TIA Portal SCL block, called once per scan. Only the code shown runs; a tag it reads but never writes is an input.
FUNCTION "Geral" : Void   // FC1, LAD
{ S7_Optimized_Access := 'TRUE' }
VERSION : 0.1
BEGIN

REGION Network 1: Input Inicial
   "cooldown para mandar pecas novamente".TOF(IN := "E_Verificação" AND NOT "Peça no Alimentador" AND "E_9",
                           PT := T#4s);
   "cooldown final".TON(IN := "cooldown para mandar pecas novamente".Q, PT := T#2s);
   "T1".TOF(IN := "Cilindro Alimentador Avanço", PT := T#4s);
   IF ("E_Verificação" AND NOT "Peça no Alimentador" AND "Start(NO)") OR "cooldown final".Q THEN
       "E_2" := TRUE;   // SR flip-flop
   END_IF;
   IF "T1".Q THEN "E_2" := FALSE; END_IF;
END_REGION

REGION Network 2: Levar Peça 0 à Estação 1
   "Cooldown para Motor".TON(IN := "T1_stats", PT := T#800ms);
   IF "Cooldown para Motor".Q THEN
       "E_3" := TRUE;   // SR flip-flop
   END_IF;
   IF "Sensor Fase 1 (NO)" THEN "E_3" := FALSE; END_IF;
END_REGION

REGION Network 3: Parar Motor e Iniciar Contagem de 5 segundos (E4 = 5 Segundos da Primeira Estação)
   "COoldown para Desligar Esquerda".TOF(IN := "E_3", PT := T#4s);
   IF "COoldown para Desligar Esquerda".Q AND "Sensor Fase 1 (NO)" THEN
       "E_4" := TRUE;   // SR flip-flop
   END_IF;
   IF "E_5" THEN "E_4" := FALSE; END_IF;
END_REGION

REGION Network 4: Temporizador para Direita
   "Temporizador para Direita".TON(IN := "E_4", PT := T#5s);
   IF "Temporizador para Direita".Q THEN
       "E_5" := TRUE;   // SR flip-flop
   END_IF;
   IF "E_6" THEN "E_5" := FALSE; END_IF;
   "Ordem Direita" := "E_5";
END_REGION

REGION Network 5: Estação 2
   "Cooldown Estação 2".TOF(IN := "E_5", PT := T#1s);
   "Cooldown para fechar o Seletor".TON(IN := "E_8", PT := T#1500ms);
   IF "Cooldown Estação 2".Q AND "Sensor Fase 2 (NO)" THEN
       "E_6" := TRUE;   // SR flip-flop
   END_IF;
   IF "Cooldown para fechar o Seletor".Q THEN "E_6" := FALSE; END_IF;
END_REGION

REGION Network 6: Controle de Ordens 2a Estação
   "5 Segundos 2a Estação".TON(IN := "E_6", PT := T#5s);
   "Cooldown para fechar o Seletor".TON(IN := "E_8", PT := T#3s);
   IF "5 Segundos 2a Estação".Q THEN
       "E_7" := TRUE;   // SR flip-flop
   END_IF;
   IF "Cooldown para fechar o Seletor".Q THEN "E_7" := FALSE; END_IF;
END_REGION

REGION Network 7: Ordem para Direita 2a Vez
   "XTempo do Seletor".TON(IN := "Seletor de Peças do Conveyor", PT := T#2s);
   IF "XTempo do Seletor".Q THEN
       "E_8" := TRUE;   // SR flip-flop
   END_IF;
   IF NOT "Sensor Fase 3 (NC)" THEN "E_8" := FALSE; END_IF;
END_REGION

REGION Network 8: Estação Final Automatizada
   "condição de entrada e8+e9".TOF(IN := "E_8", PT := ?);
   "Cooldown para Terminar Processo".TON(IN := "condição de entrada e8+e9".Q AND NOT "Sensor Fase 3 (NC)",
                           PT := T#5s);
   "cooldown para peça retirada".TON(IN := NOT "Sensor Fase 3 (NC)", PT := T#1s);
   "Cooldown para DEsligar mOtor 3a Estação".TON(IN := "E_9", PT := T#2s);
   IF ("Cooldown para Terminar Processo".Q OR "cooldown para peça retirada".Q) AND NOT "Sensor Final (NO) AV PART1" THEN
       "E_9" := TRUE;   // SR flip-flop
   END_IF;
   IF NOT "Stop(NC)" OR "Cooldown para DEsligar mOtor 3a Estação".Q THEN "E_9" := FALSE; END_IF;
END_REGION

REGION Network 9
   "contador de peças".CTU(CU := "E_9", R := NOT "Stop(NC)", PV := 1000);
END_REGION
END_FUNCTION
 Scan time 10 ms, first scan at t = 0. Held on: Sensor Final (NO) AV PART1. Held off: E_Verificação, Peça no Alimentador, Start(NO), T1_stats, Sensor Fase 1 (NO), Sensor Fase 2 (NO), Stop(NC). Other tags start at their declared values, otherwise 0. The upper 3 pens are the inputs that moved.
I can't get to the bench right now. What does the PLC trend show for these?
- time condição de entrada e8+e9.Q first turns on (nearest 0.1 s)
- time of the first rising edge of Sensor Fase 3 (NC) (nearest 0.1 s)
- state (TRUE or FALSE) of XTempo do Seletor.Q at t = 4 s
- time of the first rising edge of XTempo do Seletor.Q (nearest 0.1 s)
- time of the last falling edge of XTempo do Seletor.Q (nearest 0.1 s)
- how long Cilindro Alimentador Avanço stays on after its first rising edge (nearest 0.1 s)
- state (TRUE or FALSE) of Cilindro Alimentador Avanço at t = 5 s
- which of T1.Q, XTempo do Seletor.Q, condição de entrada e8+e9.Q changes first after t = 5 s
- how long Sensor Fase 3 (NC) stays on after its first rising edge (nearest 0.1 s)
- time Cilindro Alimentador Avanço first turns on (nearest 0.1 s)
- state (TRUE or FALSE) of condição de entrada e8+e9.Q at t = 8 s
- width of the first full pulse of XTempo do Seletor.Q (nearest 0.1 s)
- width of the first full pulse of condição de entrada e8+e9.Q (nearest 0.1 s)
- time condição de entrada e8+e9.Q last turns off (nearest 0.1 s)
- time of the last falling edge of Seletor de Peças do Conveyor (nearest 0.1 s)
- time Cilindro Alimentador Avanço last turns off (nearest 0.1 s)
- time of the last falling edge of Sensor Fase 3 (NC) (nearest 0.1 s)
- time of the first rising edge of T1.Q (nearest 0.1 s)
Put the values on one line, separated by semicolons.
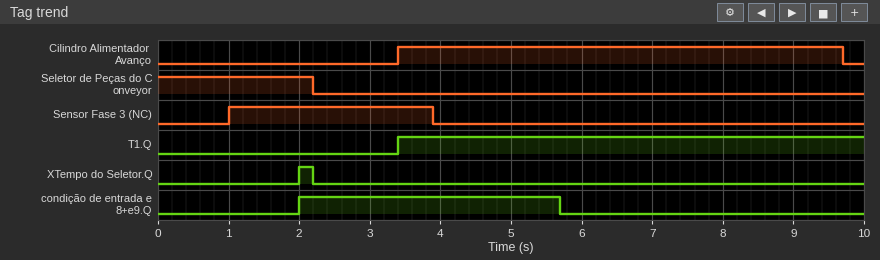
2.0 s; 1.0 s; FALSE; 2.0 s; 2.2 s; 6.3 s; TRUE; condição de entrada e8+e9.Q; 2.9 s; 3.4 s; FALSE; 0.2 s; 3.7 s; 5.7 s; 2.2 s; 9.7 s; 3.9 s; 3.4 s
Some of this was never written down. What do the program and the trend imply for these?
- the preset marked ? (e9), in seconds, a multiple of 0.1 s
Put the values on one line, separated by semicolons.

1.8 s
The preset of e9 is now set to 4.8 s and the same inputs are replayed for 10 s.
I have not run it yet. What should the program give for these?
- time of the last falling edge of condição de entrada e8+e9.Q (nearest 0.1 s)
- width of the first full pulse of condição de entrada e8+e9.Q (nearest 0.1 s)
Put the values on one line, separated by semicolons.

8.7 s; 6.7 s
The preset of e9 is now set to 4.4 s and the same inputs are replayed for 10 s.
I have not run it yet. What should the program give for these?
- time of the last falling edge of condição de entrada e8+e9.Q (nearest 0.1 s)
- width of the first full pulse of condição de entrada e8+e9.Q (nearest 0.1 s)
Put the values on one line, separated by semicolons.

8.3 s; 6.3 s
